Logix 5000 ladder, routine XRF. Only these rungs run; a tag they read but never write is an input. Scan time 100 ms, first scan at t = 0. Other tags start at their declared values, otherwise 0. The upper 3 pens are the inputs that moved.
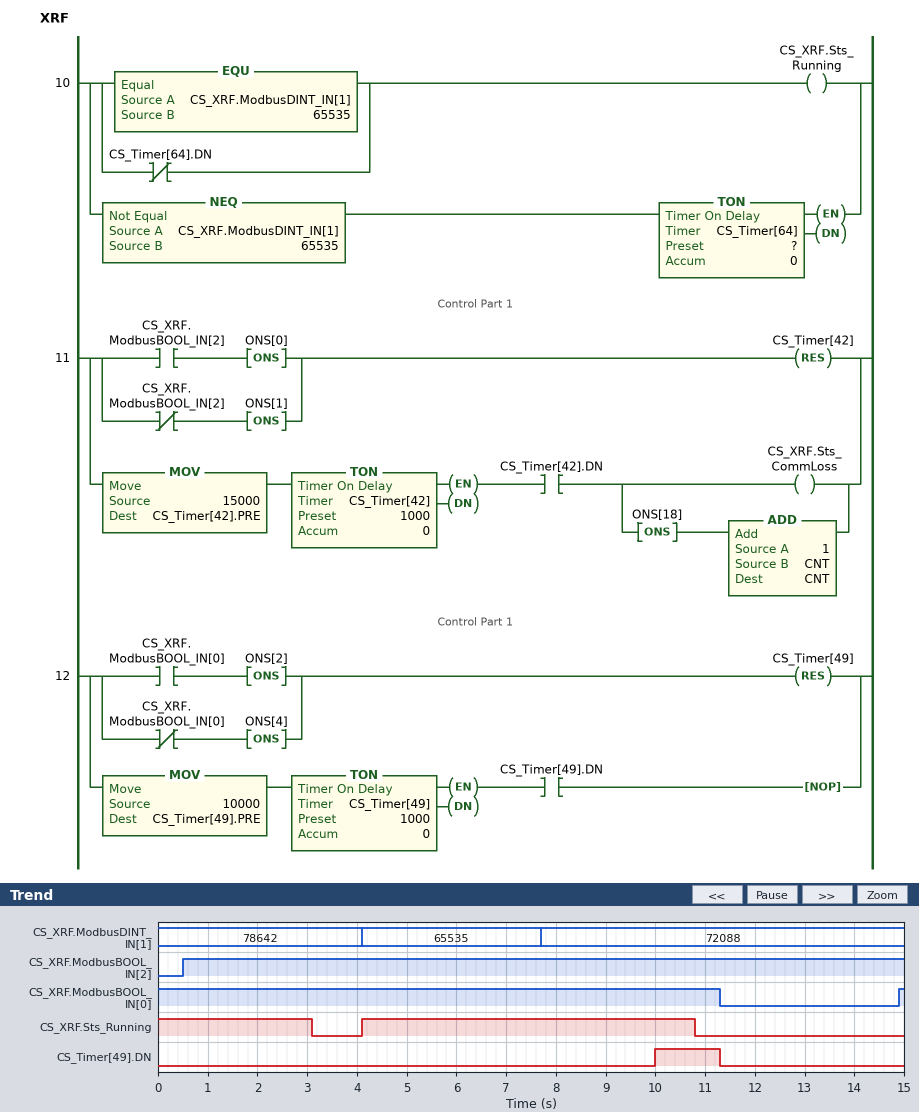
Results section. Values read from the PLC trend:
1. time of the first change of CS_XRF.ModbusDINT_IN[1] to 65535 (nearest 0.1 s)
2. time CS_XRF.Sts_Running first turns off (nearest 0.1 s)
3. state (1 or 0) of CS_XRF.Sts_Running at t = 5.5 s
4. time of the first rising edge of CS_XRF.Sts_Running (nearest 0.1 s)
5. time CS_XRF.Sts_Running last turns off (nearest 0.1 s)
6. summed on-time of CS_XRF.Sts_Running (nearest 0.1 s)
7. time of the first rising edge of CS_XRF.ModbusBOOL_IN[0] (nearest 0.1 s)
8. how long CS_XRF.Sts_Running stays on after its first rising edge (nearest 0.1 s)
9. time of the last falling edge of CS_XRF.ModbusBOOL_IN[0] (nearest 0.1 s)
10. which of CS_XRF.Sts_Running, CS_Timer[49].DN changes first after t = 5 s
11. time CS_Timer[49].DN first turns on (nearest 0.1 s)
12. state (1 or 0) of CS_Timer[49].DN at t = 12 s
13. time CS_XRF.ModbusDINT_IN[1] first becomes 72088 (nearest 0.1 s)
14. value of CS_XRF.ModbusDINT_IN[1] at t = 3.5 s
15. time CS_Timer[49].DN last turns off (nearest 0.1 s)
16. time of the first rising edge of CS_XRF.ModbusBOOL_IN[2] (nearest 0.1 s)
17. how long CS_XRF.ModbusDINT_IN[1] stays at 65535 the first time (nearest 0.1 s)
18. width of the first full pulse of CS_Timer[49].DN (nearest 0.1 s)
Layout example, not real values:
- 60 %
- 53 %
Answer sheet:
- 4.1 s
- 3.1 s
- 1
- 4.1 s
- 10.8 s
- 9.8 s
- 14.9 s
- 6.7 s
- 11.3 s
- CS_Timer[49].DN
- 10.0 s
- 0
- 7.7 s
- 78642
- 11.3 s
- 0.5 s
- 3.6 s
- 1.3 s
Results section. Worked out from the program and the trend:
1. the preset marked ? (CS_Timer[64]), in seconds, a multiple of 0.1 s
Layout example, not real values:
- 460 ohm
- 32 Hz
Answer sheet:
- 3.0 s
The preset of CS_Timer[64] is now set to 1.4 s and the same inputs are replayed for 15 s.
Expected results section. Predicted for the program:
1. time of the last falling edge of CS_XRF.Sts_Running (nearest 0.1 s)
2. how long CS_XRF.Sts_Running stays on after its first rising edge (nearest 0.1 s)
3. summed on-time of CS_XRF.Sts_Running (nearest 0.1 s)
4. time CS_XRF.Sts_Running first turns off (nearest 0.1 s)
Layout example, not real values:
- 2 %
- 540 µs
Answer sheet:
- 9.2 s
- 5.1 s
- 6.6 s
- 1.5 s
